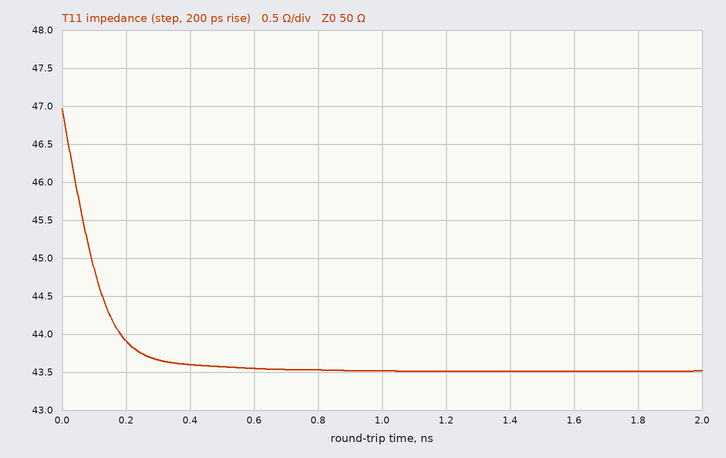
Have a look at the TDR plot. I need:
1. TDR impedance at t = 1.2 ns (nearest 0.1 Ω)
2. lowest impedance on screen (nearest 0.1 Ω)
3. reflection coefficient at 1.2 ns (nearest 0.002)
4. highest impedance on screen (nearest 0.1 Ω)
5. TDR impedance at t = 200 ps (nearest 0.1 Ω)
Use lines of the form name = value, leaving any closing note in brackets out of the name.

TDR impedance at t = 1.2 ns = 43.5 Ω
lowest impedance on screen = 43.5 Ω
reflection coefficient at 1.2 ns = -0.070
highest impedance on screen = 47.0 Ω
TDR impedance at t = 200 ps = 43.9 Ω
